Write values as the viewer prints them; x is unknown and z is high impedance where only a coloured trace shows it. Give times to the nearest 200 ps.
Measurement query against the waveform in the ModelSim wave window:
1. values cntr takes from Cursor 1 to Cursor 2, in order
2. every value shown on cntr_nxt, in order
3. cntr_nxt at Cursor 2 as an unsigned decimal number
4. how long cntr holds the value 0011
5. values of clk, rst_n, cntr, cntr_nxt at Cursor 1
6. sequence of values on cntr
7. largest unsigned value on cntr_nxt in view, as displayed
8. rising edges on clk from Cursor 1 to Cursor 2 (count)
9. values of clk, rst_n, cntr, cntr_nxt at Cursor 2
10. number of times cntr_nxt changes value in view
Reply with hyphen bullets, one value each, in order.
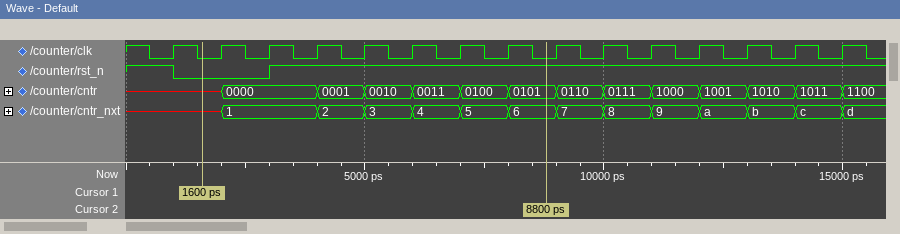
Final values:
- x, 0000, 0001, 0010, 0011, 0100, 0101
- x, 1, 2, 3, 4, 5, 6, 7, 8, 9, a, b, c, d
- 6
- 1000 ps
- clk=0, rst_n=0, cntr=x, cntr_nxt=x
- x, 0000, 0001, 0010, 0011, 0100, 0101, 0110, 0111, 1000, 1001, 1010, 1011, 1100
- d
- 7
- clk=0, rst_n=1, cntr=0101, cntr_nxt=6
- 13
